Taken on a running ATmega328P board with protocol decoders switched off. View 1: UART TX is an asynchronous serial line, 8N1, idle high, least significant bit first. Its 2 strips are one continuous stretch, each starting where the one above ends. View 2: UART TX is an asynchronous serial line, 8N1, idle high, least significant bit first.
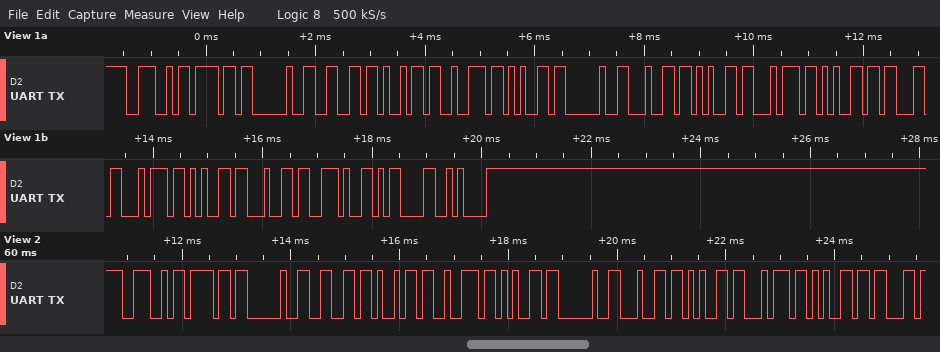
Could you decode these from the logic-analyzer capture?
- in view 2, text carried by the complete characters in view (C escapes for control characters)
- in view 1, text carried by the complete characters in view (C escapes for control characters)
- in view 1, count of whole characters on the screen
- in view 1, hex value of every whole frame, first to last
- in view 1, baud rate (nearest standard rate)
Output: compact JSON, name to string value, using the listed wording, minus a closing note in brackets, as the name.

{"in view 2, text carried by the complete characters in view": "\"No fire detec\"", "in view 1, text carried by the complete characters in view": "\"No fire detected.\\r\\n\"", "in view 1, count of whole characters on the screen": "19", "in view 1, hex value of every whole frame, first to last": "4E 6F 20 66 69 72 65 20 64 65 74 65 63 74 65 64 2E 0D 0A", "in view 1, baud rate": "9600 baud"}
